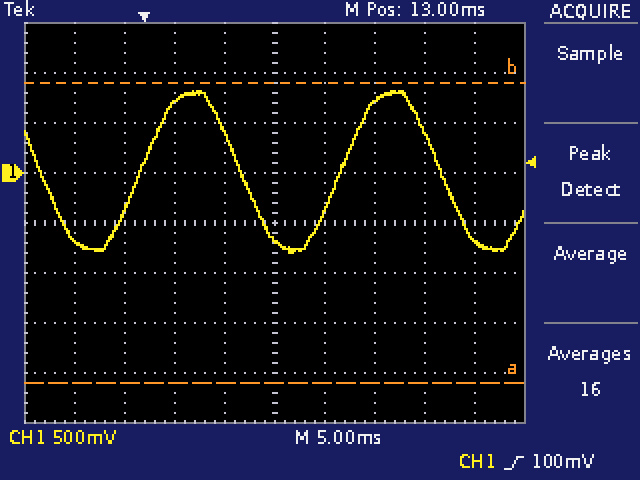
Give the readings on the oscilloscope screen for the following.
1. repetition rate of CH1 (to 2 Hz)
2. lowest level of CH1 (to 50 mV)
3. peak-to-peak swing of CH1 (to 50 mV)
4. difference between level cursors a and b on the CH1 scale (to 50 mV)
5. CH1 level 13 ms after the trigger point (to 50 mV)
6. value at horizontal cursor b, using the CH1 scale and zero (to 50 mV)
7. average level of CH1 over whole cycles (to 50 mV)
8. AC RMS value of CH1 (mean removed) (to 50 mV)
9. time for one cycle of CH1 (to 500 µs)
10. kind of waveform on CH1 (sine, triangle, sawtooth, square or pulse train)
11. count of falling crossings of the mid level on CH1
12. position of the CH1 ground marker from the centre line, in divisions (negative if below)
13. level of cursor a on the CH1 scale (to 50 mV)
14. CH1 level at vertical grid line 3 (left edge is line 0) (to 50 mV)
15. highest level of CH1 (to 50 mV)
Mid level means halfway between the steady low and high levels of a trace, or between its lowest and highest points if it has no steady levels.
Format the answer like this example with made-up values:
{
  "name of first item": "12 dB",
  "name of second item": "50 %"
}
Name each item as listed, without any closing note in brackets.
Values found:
{
  "repetition rate of CH1": "50 Hz",
  "lowest level of CH1": "-800 mV",
  "peak-to-peak swing of CH1": "1.60 V",
  "difference between level cursors a and b on the CH1 scale": "3.00 V",
  "CH1 level 13 ms after the trigger point": "-650 mV",
  "value at horizontal cursor b, using the CH1 scale and zero": "900 mV",
  "average level of CH1 over whole cycles": "0 mV",
  "AC RMS value of CH1 (mean removed)": "550 mV",
  "time for one cycle of CH1": "20.0 ms",
  "kind of waveform on CH1": "sine",
  "count of falling crossings of the mid level on CH1": "3",
  "position of the CH1 ground marker from the centre line, in divisions": "+1.0 div",
  "level of cursor a on the CH1 scale": "-2.10 V",
  "CH1 level at vertical grid line 3 (left edge is line 0)": "700 mV",
  "highest level of CH1": "800 mV"
}
